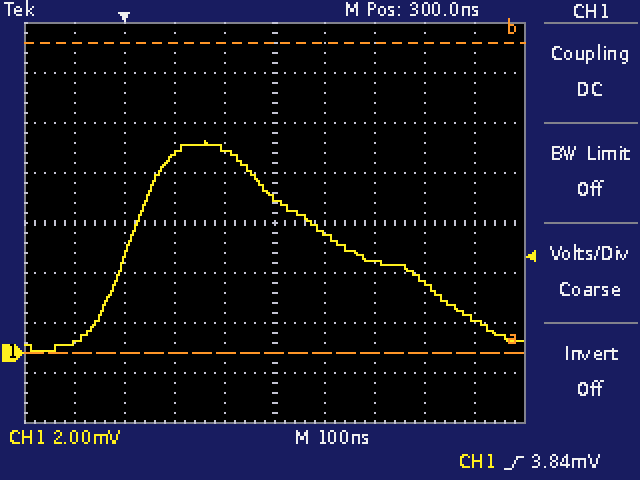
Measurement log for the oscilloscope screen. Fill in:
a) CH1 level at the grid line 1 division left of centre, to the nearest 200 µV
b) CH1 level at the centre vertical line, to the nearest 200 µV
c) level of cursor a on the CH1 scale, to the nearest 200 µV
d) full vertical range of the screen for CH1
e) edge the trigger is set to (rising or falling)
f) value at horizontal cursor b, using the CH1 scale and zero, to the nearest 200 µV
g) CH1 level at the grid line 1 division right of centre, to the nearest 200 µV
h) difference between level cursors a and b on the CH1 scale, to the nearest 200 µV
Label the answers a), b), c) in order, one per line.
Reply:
a) 8.2 mV
b) 6.2 mV
c) 0.0 mV
d) 16 mV
e) rising
f) 12.4 mV
g) 4.8 mV
h) 12.4 mV
